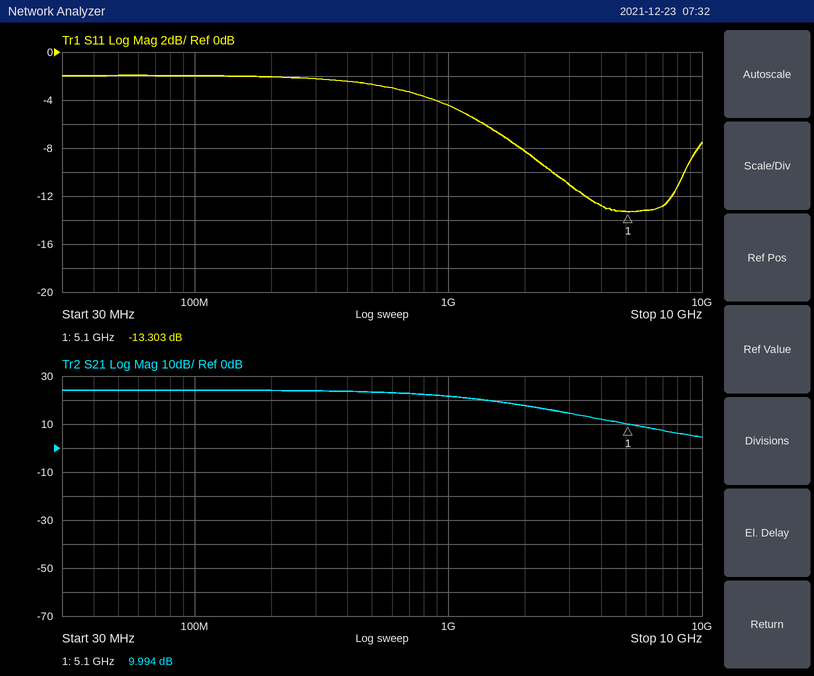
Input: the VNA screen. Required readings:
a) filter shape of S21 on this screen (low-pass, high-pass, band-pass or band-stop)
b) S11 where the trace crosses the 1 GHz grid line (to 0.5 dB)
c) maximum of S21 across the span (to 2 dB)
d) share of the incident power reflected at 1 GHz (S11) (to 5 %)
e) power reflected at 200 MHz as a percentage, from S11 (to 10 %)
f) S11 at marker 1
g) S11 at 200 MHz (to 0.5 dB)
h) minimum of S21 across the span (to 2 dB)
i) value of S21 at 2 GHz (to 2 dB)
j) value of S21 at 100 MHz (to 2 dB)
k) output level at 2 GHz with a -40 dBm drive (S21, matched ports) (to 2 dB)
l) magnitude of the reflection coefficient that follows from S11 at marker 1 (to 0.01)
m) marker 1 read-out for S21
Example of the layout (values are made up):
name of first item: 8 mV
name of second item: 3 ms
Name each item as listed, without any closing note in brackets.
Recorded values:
filter shape of S21 on this screen: low-pass
S11 where the trace crosses the 1 GHz grid line: -4.5 dB
maximum of S21 across the span: 24 dB
share of the incident power reflected at 1 GHz (S11): 35 %
power reflected at 200 MHz as a percentage, from S11: 60 %
S11 at marker 1: -13.303 dB
S11 at 200 MHz: -2.0 dB
minimum of S21 across the span: 4 dB
value of S21 at 2 GHz: 18 dB
value of S21 at 100 MHz: 24 dB
output level at 2 GHz with a -40 dBm drive (S21, matched ports): -22 dBm
magnitude of the reflection coefficient that follows from S11 at marker 1: 0.22
marker 1 read-out for S21: 9.994 dB
